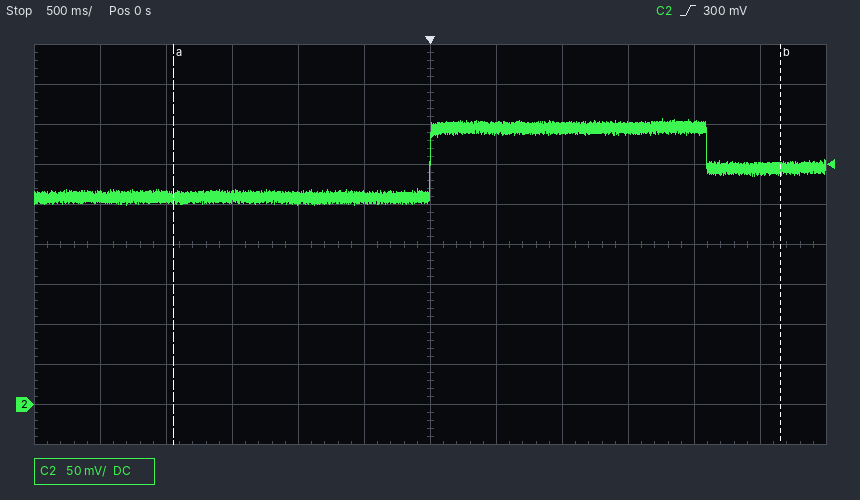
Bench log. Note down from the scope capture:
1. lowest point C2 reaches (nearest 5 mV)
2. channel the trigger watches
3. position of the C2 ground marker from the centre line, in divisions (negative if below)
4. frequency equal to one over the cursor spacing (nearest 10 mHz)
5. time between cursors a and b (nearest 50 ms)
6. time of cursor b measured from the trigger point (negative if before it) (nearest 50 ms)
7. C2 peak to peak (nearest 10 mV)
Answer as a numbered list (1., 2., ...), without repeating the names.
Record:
1. 250 mV
2. C2
3. -4.0 div
4. 220 mHz
5. 4.60 s
6. +2.65 s
7. 110 mV
